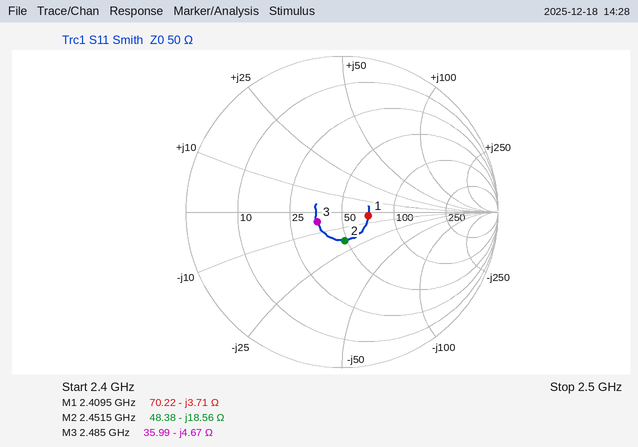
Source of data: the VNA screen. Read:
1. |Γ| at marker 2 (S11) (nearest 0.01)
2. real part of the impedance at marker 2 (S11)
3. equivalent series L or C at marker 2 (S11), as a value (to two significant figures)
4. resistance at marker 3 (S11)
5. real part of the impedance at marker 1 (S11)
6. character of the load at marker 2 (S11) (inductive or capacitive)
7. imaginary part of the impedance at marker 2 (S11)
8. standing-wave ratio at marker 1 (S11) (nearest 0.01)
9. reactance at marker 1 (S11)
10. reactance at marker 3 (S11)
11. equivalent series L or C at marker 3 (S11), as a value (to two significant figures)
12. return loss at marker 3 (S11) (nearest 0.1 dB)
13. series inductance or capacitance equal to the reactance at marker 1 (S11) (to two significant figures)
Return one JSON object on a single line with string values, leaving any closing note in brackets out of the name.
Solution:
{"|Γ| at marker 2 (S11)": "0.19", "real part of the impedance at marker 2": "48.38 Ω", "equivalent series L or C at marker 2 (S11), as a value": "3.5 pF", "resistance at marker 3": "35.99 Ω", "real part of the impedance at marker 1": "70.22 Ω", "character of the load at marker 2 (S11)": "capacitive", "imaginary part of the impedance at marker 2": "-18.56 Ω", "standing-wave ratio at marker 1 (S11)": "1.41", "reactance at marker 1": "-3.71 Ω", "reactance at marker 3": "-4.67 Ω", "equivalent series L or C at marker 3 (S11), as a value": "14 pF", "return loss at marker 3 (S11)": "15.3 dB", "series inductance or capacitance equal to the reactance at marker 1 (S11)": "18 pF"}
